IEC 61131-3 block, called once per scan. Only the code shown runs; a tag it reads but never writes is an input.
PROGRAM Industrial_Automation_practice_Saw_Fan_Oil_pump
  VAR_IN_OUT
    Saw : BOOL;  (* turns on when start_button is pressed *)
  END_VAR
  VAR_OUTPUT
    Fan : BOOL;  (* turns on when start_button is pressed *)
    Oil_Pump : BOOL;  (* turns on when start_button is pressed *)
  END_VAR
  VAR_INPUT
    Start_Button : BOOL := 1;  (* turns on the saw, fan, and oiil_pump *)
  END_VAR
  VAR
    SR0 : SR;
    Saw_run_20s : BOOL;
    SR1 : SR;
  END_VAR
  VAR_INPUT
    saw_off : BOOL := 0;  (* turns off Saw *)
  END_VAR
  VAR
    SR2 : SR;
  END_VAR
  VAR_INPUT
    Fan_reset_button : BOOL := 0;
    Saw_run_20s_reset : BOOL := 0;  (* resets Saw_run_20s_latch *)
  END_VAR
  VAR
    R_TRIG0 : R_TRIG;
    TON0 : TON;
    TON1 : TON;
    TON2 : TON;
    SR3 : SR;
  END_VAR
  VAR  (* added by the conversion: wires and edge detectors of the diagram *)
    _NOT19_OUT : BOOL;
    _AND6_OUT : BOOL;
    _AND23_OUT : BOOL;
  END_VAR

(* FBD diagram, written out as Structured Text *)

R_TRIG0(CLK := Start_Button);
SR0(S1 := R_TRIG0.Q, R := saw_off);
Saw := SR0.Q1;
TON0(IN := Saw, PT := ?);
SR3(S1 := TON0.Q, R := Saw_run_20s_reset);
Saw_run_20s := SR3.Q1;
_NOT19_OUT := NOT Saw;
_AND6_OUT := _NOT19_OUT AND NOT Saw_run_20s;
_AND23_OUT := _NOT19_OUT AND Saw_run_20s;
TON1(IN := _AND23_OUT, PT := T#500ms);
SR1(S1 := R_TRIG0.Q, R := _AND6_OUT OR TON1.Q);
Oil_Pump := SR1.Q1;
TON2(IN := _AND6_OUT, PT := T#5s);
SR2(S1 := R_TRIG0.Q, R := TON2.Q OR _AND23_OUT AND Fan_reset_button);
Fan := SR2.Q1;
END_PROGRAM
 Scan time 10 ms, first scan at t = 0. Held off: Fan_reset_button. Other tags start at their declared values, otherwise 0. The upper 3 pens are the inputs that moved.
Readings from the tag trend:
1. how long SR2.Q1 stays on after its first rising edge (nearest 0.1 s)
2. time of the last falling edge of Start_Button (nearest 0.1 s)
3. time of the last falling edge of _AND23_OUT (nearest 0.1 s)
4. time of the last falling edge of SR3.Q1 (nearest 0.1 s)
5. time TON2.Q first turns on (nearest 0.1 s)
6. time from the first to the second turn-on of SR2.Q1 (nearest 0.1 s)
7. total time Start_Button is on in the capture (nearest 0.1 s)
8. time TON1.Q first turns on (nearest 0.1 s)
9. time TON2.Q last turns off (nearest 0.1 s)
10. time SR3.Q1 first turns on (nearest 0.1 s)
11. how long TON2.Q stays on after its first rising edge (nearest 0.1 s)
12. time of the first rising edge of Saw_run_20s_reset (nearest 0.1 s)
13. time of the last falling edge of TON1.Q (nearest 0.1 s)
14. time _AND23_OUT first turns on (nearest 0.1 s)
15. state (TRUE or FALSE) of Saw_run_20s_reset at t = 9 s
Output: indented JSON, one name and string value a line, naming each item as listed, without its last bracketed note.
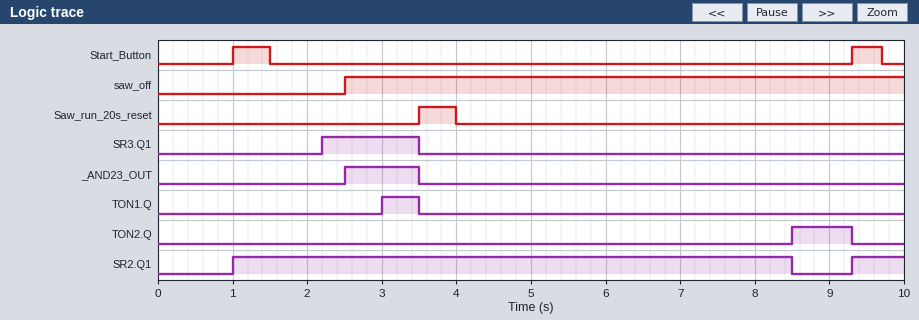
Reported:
{
  "how long SR2.Q1 stays on after its first rising edge": "7.5 s",
  "time of the last falling edge of Start_Button": "9.7 s",
  "time of the last falling edge of _AND23_OUT": "3.5 s",
  "time of the last falling edge of SR3.Q1": "3.5 s",
  "time TON2.Q first turns on": "8.5 s",
  "time from the first to the second turn-on of SR2.Q1": "8.3 s",
  "total time Start_Button is on in the capture": "0.9 s",
  "time TON1.Q first turns on": "3.0 s",
  "time TON2.Q last turns off": "9.3 s",
  "time SR3.Q1 first turns on": "2.2 s",
  "how long TON2.Q stays on after its first rising edge": "0.8 s",
  "time of the first rising edge of Saw_run_20s_reset": "3.5 s",
  "time of the last falling edge of TON1.Q": "3.5 s",
  "time _AND23_OUT first turns on": "2.5 s",
  "state (TRUE or FALSE) of Saw_run_20s_reset at t = 9 s": "FALSE"
}
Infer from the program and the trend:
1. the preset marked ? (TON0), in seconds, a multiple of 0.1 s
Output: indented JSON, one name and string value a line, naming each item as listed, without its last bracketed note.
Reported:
{
  "the preset marked ? (TON0), in seconds, a multiple of 0.1 s": "1.2 s"
}
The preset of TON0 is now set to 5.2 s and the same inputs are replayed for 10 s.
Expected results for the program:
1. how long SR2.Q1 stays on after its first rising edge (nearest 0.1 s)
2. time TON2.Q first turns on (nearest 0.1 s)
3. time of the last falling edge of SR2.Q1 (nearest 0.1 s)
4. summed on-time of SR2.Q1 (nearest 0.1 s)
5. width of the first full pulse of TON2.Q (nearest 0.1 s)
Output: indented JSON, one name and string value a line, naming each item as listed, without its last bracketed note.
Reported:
{
  "how long SR2.Q1 stays on after its first rising edge": "6.5 s",
  "time TON2.Q first turns on": "7.5 s",
  "time of the last falling edge of SR2.Q1": "7.5 s",
  "summed on-time of SR2.Q1": "7.2 s",
  "width of the first full pulse of TON2.Q": "1.8 s"
}
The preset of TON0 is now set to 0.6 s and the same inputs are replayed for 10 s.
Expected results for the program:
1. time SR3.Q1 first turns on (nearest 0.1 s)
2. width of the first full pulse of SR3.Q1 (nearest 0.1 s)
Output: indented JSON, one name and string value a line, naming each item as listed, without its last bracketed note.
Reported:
{
  "time SR3.Q1 first turns on": "1.6 s",
  "width of the first full pulse of SR3.Q1": "1.9 s"
}
